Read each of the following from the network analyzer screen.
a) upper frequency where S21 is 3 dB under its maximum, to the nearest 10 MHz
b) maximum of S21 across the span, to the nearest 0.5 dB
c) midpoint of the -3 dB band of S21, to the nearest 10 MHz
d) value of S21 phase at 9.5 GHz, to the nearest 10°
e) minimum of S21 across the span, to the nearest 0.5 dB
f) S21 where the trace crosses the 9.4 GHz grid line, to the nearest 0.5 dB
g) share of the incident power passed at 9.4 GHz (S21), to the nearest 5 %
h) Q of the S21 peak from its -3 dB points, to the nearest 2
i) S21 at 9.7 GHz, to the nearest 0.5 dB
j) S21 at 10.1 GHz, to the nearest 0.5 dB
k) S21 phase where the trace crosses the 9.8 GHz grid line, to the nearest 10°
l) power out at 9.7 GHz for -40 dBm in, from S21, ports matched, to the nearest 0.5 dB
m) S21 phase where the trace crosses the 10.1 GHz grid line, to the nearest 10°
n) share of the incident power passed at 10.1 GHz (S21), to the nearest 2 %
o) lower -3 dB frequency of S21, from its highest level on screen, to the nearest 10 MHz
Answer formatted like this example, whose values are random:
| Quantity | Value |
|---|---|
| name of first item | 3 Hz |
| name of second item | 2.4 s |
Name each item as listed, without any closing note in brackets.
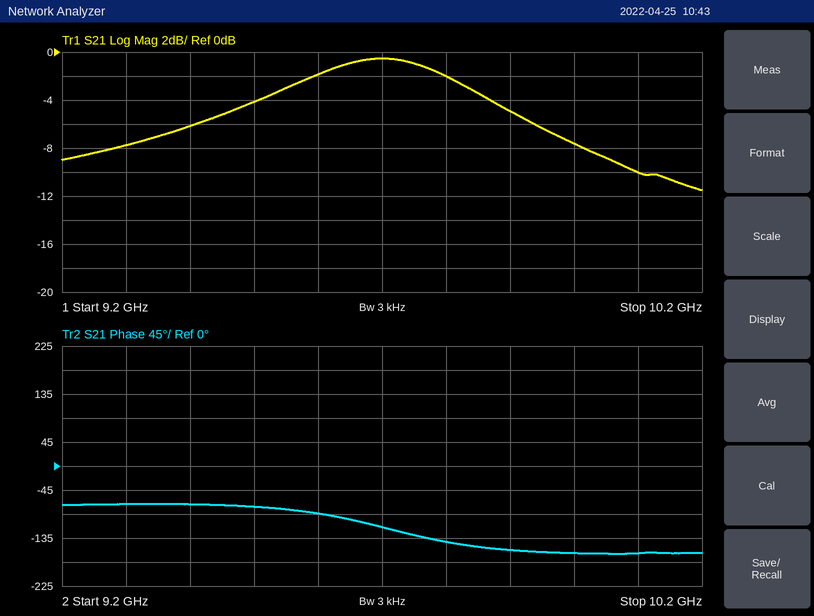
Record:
| Quantity | Value |
|---|---|
| upper frequency where S21 is 3 dB under its maximum, to the nearest 10 MHz | 9.85 GHz |
| maximum of S21 across the span, to the nearest 0.5 dB | -0.5 dB |
| midpoint of the -3 dB band of S21, to the nearest 10 MHz | 9.69 GHz |
| value of S21 phase at 9.5 GHz, to the nearest 10° | -80° |
| minimum of S21 across the span, to the nearest 0.5 dB | -11.5 dB |
| S21 where the trace crosses the 9.4 GHz grid line, to the nearest 0.5 dB | -6.0 dB |
| share of the incident power passed at 9.4 GHz (S21), to the nearest 5 % | 25 % |
| Q of the S21 peak from its -3 dB points, to the nearest 2 | 30 |
| S21 at 9.7 GHz, to the nearest 0.5 dB | -0.5 dB |
| S21 at 10.1 GHz, to the nearest 0.5 dB | -10.0 dB |
| S21 phase where the trace crosses the 9.8 GHz grid line, to the nearest 10° | -140° |
| power out at 9.7 GHz for -40 dBm in, from S21, ports matched, to the nearest 0.5 dB | -40.5 dBm |
| S21 phase where the trace crosses the 10.1 GHz grid line, to the nearest 10° | -160° |
| share of the incident power passed at 10.1 GHz (S21), to the nearest 2 % | 10 % |
| lower -3 dB frequency of S21, from its highest level on screen, to the nearest 10 MHz | 9.53 GHz |
